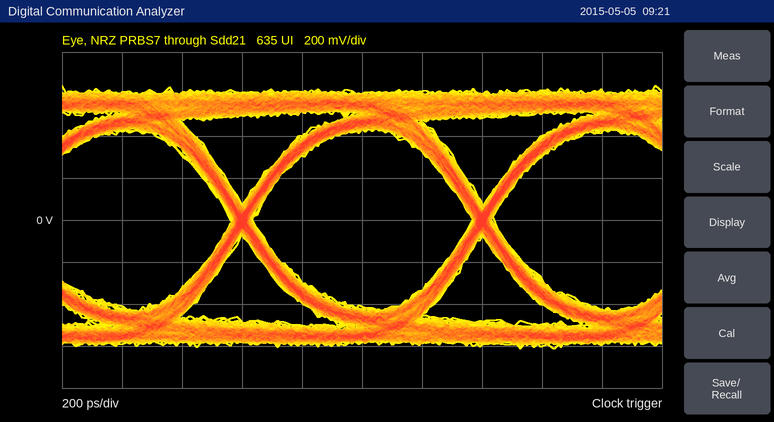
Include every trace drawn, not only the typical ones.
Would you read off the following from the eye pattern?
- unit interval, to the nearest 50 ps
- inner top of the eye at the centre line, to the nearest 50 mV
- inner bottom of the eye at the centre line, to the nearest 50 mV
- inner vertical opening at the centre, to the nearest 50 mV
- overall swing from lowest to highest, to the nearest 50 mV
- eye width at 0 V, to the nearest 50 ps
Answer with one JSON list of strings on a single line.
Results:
["800 ps", "450 mV", "-400 mV", "850 mV", "1.25 V", "750 ps"]
